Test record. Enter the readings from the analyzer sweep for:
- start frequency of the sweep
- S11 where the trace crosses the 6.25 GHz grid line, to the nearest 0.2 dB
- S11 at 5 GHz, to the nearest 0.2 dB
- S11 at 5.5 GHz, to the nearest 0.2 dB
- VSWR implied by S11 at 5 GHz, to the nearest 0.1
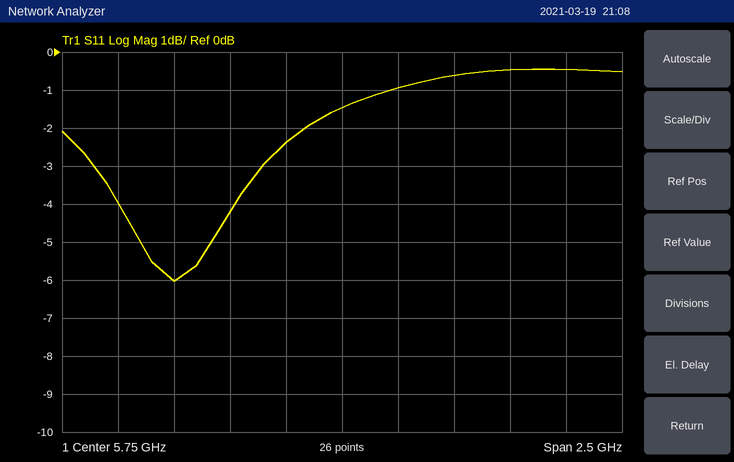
4.5 GHz
-0.6 dB
-6.0 dB
-2.4 dB
3.0
